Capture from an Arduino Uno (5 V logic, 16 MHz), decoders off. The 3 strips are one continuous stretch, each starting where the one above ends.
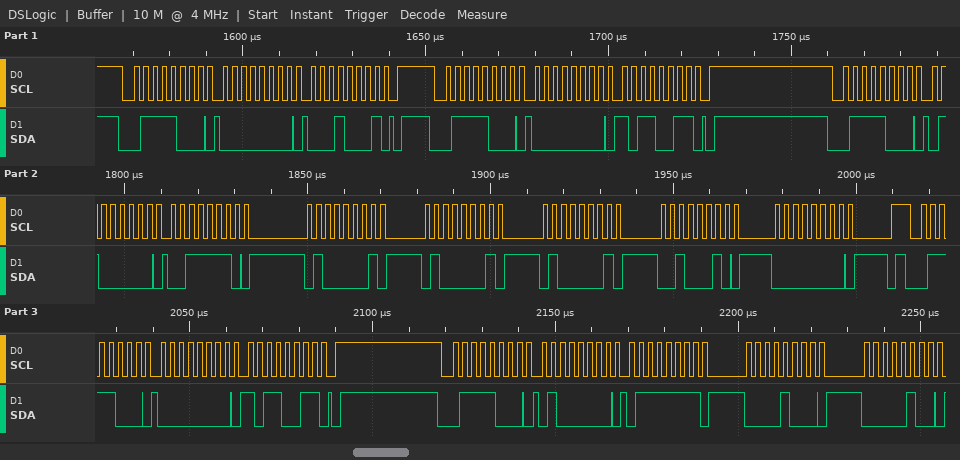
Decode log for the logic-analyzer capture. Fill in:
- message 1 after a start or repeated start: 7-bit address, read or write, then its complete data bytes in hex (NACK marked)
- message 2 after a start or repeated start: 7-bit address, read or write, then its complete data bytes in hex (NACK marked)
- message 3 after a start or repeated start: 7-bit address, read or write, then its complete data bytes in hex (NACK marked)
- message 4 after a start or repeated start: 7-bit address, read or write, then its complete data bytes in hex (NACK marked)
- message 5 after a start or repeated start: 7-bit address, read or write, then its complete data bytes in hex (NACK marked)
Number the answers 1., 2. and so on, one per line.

1. 0x3C write: 00 11
2. 0x3C write: 00 B3
3. 0x3C write: 40 3E 41 41 41 22 00
4. 0x3C write: 00 B3
5. 0x3C write: 40 7F 08 04
